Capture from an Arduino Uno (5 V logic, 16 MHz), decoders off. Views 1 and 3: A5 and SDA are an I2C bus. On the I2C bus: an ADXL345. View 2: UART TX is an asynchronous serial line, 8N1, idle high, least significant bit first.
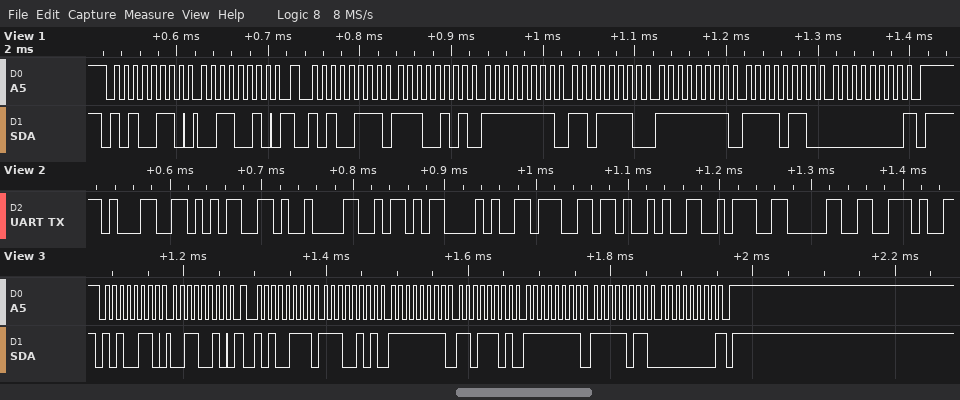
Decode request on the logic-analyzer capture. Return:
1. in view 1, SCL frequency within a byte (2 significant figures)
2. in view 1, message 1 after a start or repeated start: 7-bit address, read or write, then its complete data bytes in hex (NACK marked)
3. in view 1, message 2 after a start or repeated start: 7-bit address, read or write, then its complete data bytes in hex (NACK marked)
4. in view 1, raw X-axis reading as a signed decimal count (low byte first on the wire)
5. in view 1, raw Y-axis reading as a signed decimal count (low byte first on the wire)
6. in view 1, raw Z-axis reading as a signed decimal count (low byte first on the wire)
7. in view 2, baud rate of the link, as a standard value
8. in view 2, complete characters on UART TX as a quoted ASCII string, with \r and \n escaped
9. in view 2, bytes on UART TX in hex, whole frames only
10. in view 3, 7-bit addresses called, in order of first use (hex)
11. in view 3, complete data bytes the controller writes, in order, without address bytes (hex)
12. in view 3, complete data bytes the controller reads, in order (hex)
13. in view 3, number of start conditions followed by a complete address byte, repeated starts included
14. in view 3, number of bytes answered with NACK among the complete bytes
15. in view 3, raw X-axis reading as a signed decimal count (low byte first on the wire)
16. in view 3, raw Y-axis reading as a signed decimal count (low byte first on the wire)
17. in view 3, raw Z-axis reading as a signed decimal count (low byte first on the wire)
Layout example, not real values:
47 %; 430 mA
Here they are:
100 kHz; 0x53 write: 32; 0x53 read: E5 FF DE FF F6 00 NACK; -27; -34; 246; 115200 baud; "15\tZ(g):0."; 31 35 09 5A 28 67 29 3A 30 2E; 0x53; 32; E5 FF DD FF FB 00; 2; 1; -27; -35; 251
